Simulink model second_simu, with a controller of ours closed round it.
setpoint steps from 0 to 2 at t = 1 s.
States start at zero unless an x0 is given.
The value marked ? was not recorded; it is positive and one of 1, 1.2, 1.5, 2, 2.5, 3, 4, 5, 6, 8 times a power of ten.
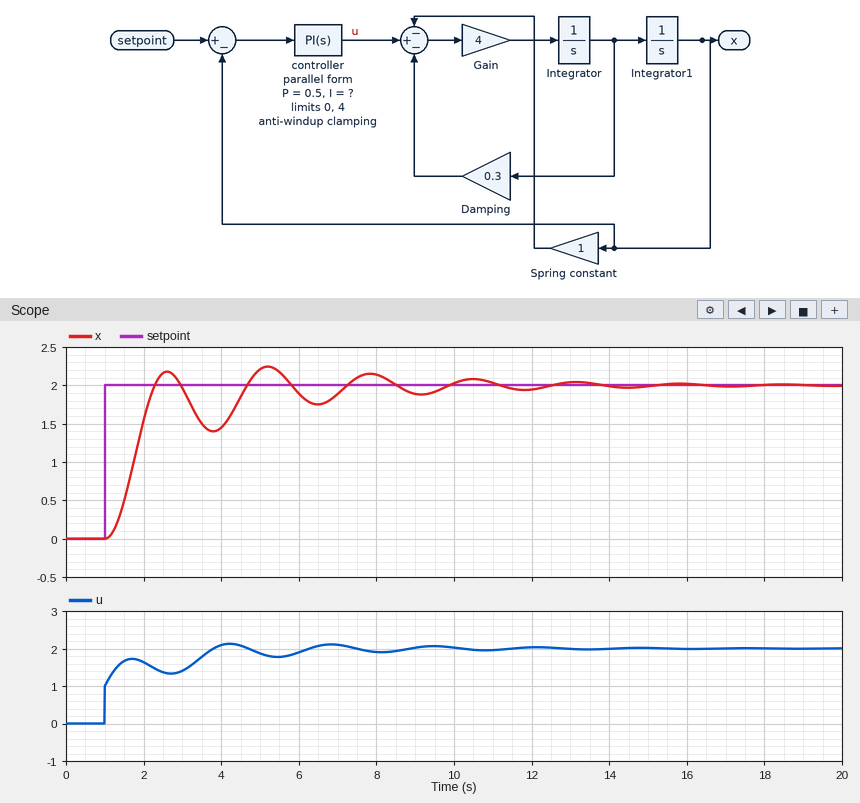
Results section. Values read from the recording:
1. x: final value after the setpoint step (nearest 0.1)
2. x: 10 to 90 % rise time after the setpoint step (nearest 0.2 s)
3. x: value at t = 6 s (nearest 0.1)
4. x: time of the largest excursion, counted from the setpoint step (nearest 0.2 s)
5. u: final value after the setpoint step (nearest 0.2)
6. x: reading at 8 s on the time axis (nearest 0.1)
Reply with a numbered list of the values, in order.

1. 2.0
2. 0.8 s
3. 1.9
4. 4.2 s
5. 2.0
6. 2.1
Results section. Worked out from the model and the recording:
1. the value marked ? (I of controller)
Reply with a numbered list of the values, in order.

1. 1
